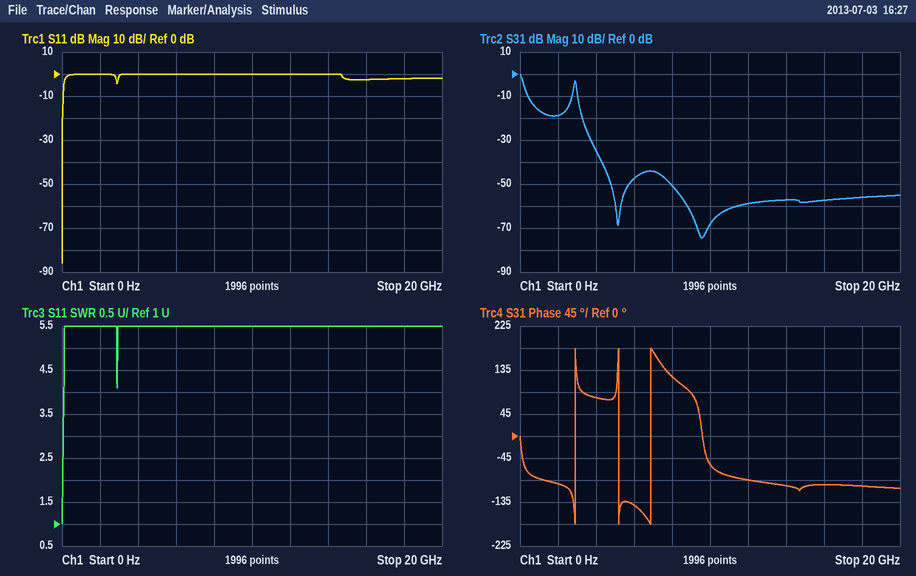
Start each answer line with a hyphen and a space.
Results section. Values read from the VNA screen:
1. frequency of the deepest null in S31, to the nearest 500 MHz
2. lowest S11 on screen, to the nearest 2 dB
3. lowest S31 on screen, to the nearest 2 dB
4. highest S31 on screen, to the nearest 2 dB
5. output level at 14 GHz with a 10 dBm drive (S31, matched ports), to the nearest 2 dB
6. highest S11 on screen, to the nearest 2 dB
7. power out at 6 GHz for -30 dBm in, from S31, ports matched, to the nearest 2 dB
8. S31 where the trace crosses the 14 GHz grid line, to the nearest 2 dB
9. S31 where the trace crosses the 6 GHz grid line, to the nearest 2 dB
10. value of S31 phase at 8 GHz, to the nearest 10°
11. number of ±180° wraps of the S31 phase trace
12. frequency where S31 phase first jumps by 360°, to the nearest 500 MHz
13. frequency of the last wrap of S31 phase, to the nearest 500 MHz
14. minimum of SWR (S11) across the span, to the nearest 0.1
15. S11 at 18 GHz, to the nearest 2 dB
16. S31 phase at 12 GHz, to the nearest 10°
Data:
- 9.5 GHz
- -86 dB
- -74 dB
- 0 dB
- -48 dBm
- 0 dB
- -78 dBm
- -58 dB
- -48 dB
- 120°
- 3
- 3.0 GHz
- 7.0 GHz
- 1.0
- -2 dB
- -90°
